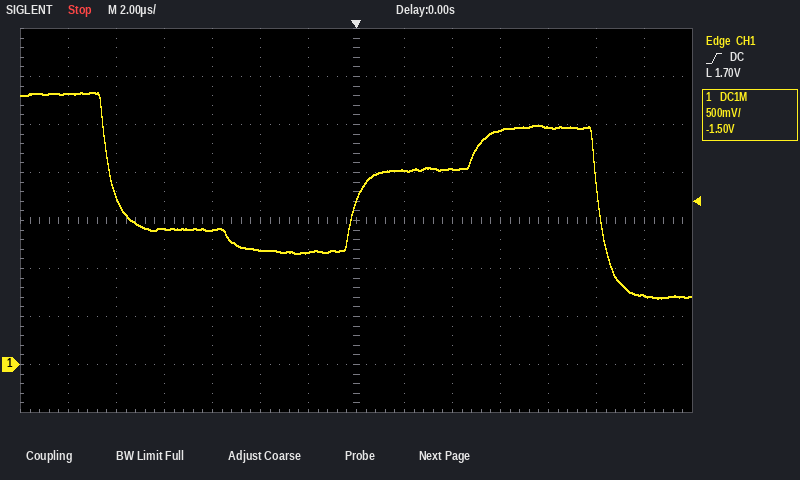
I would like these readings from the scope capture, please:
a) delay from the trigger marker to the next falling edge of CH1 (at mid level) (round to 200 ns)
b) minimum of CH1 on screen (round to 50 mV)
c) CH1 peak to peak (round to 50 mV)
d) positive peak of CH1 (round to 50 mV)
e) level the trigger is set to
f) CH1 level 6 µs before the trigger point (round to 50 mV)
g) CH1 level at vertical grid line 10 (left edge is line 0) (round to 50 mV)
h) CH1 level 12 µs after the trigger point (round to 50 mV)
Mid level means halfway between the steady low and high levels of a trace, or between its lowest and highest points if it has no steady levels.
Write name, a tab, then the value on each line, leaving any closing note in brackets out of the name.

delay from the trigger marker to the next falling edge of CH1 (at mid level)	10.0 µs
minimum of CH1 on screen	700 mV
CH1 peak to peak	2.15 V
positive peak of CH1	2.85 V
level the trigger is set to	1.70 V
CH1 level 6 µs before the trigger point	1.40 V
CH1 level at vertical grid line 10 (left edge is line 0)	2.45 V
CH1 level 12 µs after the trigger point	700 mV
